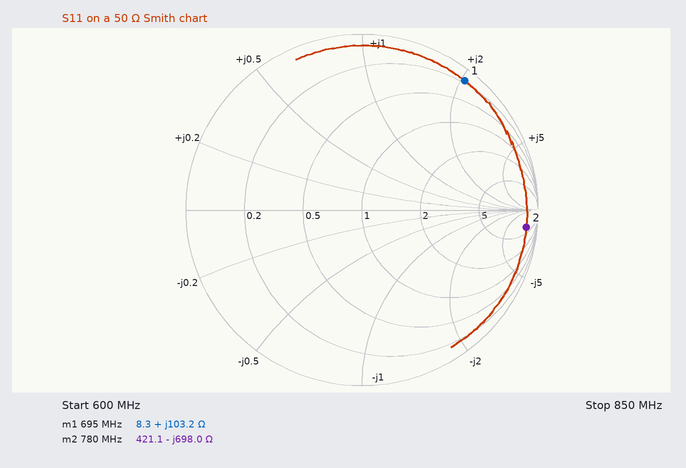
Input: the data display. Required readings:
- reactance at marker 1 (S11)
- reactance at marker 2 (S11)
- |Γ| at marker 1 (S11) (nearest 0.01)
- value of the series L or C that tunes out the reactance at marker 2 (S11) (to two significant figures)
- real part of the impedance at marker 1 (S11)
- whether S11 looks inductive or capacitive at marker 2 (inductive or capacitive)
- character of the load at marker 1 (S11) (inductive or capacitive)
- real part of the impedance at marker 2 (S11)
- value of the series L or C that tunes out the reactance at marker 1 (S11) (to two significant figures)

+103.2 Ω
-698.0 Ω
0.94
140 nH
8.3 Ω
capacitive
inductive
421.1 Ω
2.2 pF
